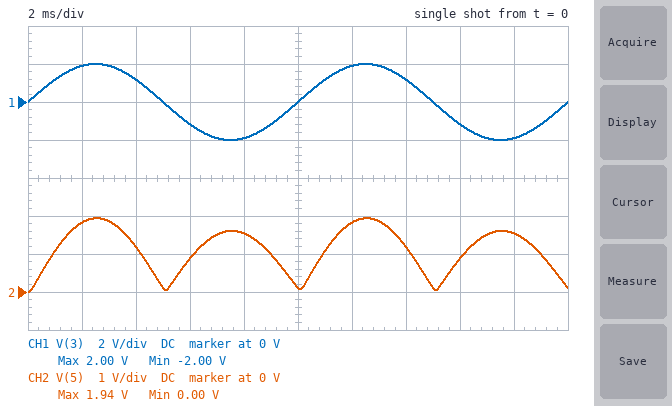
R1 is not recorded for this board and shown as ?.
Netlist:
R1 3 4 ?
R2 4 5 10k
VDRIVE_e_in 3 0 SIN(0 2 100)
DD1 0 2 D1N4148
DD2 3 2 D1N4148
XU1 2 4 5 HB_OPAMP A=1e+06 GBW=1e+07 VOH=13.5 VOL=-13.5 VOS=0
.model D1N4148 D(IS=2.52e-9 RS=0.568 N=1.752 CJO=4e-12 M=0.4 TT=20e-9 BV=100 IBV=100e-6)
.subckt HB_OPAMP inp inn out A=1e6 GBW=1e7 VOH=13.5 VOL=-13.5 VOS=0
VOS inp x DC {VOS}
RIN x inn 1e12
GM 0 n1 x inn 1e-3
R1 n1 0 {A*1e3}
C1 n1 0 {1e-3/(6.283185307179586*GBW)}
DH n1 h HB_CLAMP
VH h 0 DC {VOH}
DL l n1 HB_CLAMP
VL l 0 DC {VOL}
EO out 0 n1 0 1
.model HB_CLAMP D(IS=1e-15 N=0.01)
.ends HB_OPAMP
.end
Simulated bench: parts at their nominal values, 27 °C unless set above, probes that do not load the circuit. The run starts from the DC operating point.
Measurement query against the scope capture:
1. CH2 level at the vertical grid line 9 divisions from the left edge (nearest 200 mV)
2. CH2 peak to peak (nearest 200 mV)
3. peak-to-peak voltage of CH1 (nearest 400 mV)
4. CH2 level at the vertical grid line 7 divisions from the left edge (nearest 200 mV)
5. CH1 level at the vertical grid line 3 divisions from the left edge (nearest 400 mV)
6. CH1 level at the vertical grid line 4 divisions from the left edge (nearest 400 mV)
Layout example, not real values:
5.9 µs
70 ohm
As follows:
1.6 V
2.0 V
4.0 V
1.2 V
-1.2 V
-2.0 V
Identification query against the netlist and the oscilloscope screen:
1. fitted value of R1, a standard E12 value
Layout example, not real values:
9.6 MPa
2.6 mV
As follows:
12 kΩ
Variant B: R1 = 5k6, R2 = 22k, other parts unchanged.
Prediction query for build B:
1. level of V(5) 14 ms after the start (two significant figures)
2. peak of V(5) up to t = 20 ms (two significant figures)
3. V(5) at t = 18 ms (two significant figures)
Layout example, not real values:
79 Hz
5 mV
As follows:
1.2 V
7.7 V
7.4 V
